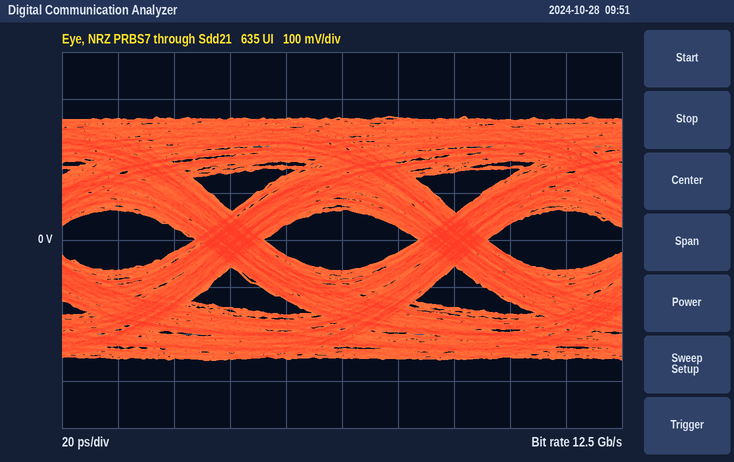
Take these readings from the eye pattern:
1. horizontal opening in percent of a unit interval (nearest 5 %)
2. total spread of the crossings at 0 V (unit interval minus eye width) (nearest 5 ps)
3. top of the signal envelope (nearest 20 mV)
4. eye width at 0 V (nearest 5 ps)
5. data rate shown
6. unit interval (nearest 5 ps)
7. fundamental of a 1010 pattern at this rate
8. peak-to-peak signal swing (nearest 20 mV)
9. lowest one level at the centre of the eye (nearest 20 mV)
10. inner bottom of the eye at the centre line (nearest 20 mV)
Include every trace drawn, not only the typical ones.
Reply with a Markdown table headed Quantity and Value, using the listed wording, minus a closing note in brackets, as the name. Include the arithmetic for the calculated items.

| Quantity | Value |
|---|---|
| horizontal opening in percent of a unit interval | 55 ps / 80 ps ≈ 68.8 %, so 70 % to the nearest 5 % |
| total spread of the crossings at 0 V (unit interval minus eye width) | 25 ps |
| top of the signal envelope | 260 mV |
| eye width at 0 V | 55 ps |
| data rate shown | 12.5 Gb/s |
| unit interval | 80 ps |
| fundamental of a 1010 pattern at this rate | 6.25 GHz |
| peak-to-peak signal swing | 520 mV |
| lowest one level at the centre of the eye | 60 mV |
| inner bottom of the eye at the centre line | -60 mV |
